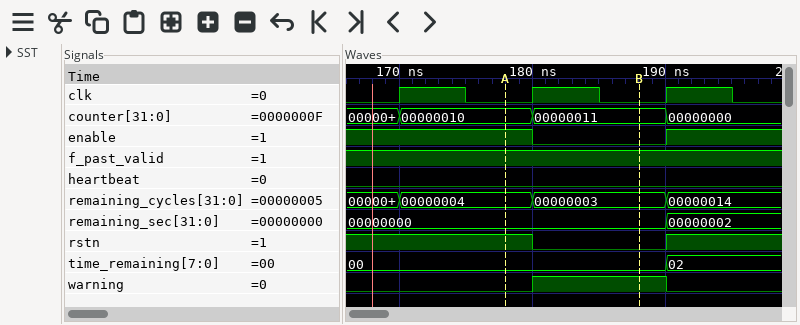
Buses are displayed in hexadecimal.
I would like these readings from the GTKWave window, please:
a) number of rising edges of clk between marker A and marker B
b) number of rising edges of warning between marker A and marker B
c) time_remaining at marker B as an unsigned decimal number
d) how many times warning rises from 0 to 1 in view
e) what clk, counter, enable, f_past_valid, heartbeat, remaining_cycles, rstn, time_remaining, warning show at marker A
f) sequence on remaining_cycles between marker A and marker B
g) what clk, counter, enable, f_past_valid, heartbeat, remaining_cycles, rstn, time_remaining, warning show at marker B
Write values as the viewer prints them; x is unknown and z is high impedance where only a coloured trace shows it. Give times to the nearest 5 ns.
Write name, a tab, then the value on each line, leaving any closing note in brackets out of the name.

number of rising edges of clk between marker A and marker B	1
number of rising edges of warning between marker A and marker B	1
time_remaining at marker B as an unsigned decimal number	0
how many times warning rises from 0 to 1 in view	1
what clk, counter, enable, f_past_valid, heartbeat, remaining_cycles, rstn, time_remaining, warning show at marker A	clk=0, counter=00000010, enable=1, f_past_valid=1, heartbeat=0, remaining_cycles=00000004, rstn=1, time_remaining=00, warning=0
sequence on remaining_cycles between marker A and marker B	00000004, 00000003
what clk, counter, enable, f_past_valid, heartbeat, remaining_cycles, rstn, time_remaining, warning show at marker B	clk=0, counter=00000011, enable=0, f_past_valid=1, heartbeat=0, remaining_cycles=00000003, rstn=0, time_remaining=00, warning=1
